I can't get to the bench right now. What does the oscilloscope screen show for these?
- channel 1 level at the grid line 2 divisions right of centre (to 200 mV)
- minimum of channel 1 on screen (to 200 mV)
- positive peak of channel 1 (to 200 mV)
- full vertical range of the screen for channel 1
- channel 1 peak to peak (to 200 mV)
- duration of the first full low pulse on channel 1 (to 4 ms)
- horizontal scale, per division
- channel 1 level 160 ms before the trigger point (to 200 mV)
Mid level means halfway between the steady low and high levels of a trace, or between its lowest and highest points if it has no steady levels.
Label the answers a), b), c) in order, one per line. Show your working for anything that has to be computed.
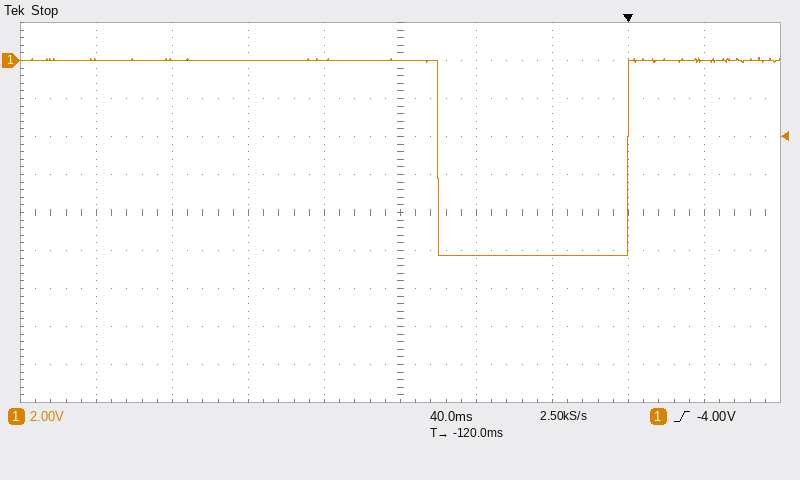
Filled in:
a) -10.2 V
b) -10.2 V
c) 200 mV
d) 20 V
e) 200 mV − (-10.2 V) = 10.4 V
f) 100 ms
g) 40 ms
h) 0.0 V
